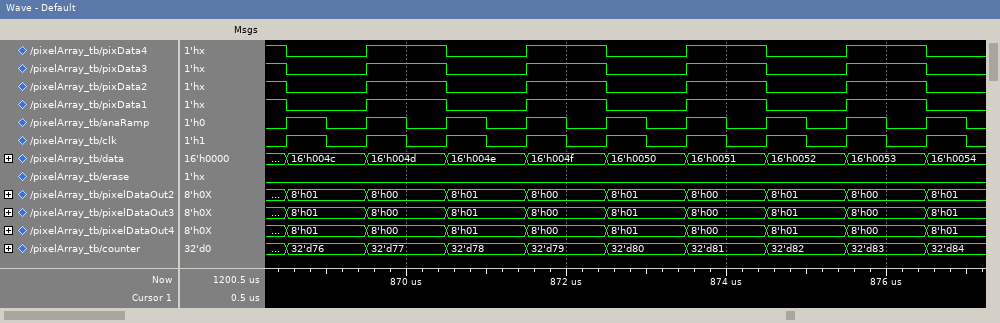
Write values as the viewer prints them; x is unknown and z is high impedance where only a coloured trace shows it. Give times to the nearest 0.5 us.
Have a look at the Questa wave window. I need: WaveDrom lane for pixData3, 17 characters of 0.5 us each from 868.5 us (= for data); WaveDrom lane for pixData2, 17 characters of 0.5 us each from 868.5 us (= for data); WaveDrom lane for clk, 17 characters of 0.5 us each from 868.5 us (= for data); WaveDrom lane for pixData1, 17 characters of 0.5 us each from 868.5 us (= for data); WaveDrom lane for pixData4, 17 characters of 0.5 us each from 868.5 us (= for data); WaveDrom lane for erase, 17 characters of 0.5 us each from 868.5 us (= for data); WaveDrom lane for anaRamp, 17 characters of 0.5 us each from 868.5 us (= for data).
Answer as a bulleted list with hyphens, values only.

- {name: 'pixData3', wave: '0.1.0.1.0.1.0.1.0'}
- {name: 'pixData2', wave: '0.1.0.1.0.1.0.1.0'}
- {name: 'clk', wave: '10101010101010101'}
- {name: 'pixData1', wave: '0.1.0.1.0.1.0.1.0'}
- {name: 'pixData4', wave: '0.1.0.1.0.1.0.1.0'}
- {name: 'erase', wave: '0................'}
- {name: 'anaRamp', wave: '10101010101010101'}
